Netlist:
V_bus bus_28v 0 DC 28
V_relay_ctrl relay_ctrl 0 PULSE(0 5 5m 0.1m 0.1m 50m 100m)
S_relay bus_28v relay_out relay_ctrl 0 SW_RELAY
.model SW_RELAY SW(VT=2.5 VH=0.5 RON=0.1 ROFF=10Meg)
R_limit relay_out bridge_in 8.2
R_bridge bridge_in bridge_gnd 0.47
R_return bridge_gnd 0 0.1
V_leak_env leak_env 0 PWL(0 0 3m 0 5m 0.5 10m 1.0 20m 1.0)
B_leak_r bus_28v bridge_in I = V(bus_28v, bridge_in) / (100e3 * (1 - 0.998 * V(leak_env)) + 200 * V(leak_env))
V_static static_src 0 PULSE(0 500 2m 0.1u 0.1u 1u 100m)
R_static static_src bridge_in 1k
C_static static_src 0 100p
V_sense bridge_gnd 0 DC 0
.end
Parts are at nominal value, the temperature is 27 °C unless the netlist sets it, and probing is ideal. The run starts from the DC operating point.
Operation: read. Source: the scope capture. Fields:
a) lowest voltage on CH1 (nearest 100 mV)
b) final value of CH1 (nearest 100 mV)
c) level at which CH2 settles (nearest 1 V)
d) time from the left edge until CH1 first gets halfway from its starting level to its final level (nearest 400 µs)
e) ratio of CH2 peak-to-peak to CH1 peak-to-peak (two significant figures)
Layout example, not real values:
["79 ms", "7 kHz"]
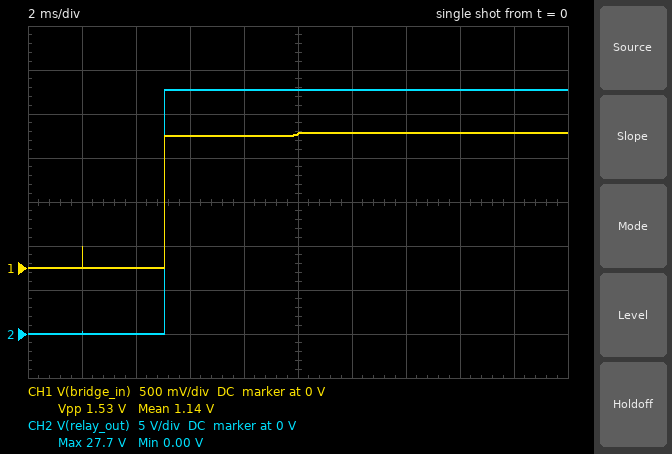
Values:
["0 V", "1.5 V", "28 V", "5.2 ms", "18"]
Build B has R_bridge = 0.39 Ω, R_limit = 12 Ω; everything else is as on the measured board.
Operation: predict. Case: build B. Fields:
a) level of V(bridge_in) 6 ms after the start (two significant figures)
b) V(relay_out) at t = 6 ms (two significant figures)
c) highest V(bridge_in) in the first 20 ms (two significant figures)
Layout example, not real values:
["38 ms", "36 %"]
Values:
["870 mV", "28 V", "900 mV"]
